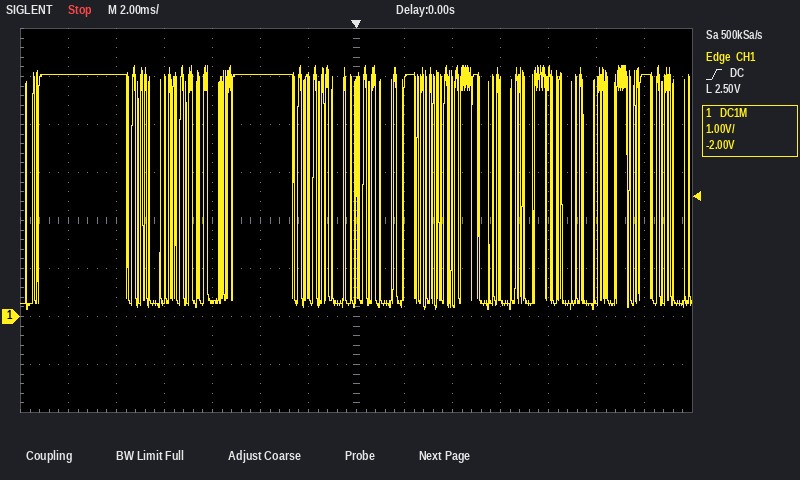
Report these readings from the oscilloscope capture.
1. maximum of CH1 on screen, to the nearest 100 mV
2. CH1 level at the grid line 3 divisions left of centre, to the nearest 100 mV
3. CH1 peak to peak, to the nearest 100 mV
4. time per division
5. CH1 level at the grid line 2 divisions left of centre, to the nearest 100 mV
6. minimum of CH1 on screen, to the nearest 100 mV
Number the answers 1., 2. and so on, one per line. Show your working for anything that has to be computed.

1. 5.2 V
2. 300 mV
3. 5.2 V − (100 mV) = 5.1 V
4. 2 ms
5. 5.0 V
6. 100 mV
